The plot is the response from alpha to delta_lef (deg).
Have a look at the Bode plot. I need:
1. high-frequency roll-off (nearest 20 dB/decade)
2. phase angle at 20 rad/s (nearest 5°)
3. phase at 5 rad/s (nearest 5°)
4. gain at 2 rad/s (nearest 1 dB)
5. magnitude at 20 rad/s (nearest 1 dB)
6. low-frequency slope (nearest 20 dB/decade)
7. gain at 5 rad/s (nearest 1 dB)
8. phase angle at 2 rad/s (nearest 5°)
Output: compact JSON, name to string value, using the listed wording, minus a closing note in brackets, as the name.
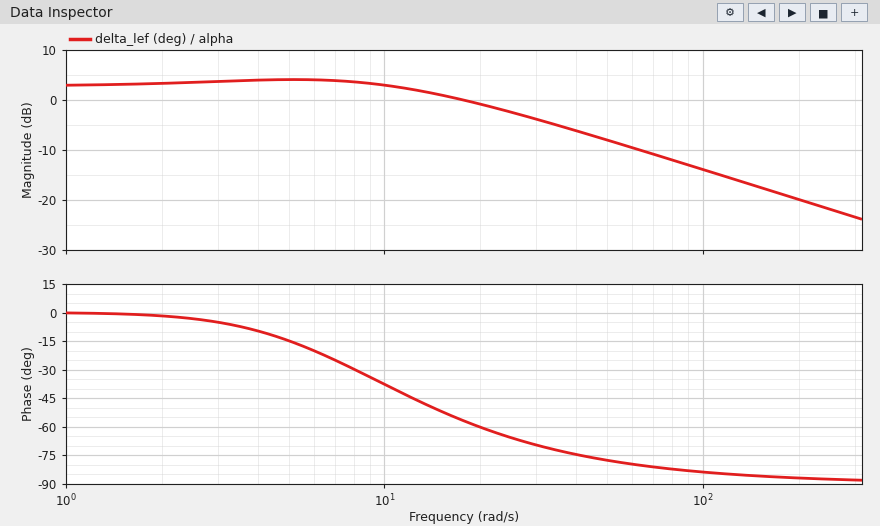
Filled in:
{"high-frequency roll-off": "-20 dB/decade", "phase angle at 20 rad/s": "-60°", "phase at 5 rad/s": "-15°", "gain at 2 rad/s": "3 dB", "magnitude at 20 rad/s": "-1 dB", "low-frequency slope": "0 dB/decade", "gain at 5 rad/s": "4 dB", "phase angle at 2 rad/s": "0°"}
